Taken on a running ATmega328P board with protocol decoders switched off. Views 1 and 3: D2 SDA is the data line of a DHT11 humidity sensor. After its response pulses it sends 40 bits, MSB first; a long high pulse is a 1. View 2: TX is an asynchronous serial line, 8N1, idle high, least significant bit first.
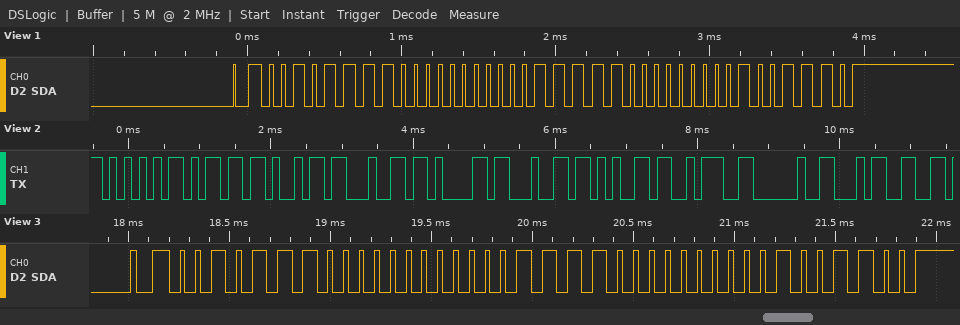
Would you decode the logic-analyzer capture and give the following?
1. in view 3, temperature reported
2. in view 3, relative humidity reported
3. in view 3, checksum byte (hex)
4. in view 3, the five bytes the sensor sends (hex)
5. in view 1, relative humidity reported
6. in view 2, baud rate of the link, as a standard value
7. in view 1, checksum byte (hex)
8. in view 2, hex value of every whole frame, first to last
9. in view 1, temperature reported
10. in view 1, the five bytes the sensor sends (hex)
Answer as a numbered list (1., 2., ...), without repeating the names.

1. 30.0 °C
2. 46 %
3. 0x4C
4. 2E 00 1E 00 4C
5. 47 %
6. 9600 baud
7. 0x4E
8. 55 6D 69 64 61 64 65 3A 20 34
9. 31.0 °C
10. 2F 00 1F 00 4E
